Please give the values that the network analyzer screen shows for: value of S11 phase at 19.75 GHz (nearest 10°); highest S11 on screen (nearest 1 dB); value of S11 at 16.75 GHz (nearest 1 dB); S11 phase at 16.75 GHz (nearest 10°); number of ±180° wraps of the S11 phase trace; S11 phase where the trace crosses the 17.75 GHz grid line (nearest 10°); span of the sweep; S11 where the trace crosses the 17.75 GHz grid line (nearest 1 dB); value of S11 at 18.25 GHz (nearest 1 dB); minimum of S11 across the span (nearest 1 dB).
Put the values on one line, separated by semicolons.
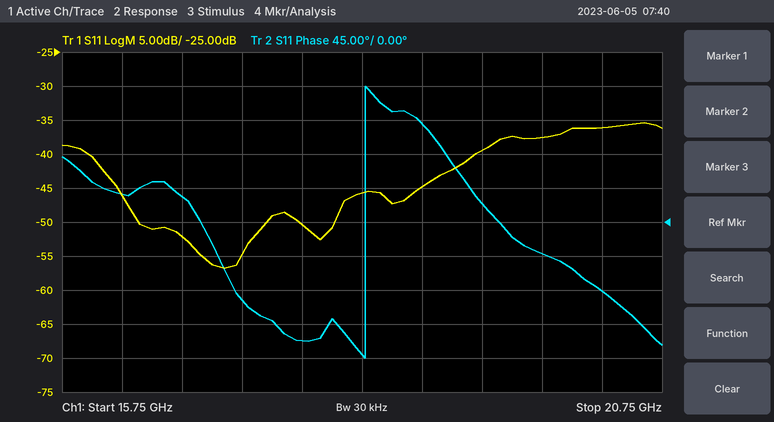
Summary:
-40°; -35 dB; -52 dB; 30°; 1; -160°; 5 GHz; -50 dB; -46 dB; -57 dB
